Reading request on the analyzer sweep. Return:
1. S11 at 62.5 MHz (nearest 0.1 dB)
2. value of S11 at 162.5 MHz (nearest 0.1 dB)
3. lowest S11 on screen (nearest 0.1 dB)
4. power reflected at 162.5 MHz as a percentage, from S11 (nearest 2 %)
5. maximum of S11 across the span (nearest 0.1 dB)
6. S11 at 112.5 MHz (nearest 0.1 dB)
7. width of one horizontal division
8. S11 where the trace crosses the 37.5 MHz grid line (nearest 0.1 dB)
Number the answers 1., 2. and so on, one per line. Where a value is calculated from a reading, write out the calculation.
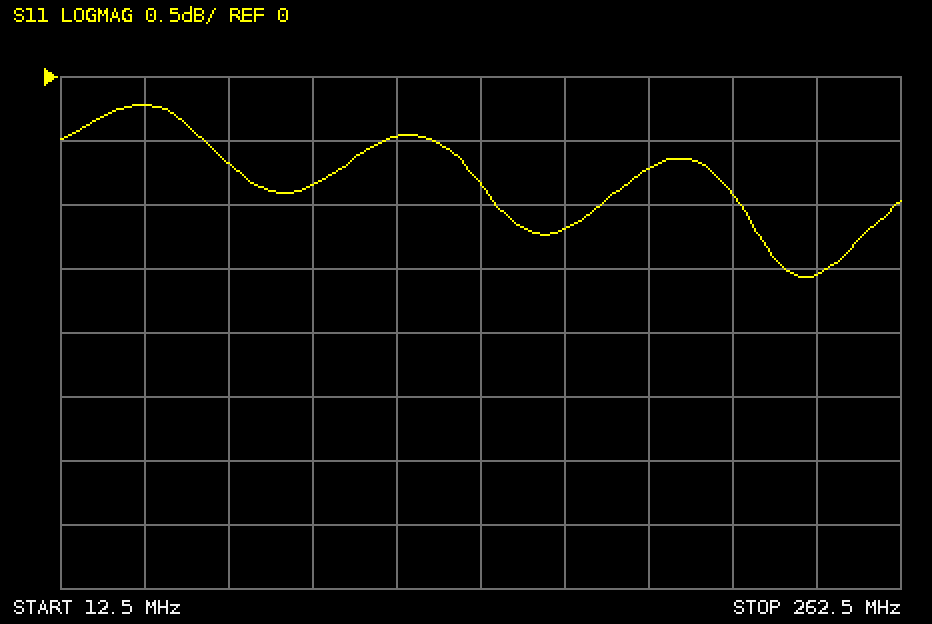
1. -0.7 dB
2. -1.2 dB
3. -1.6 dB
4. 10^(-1.2/10) ≈ 76 %
5. -0.2 dB
6. -0.5 dB
7. 25 MHz
8. -0.2 dB
